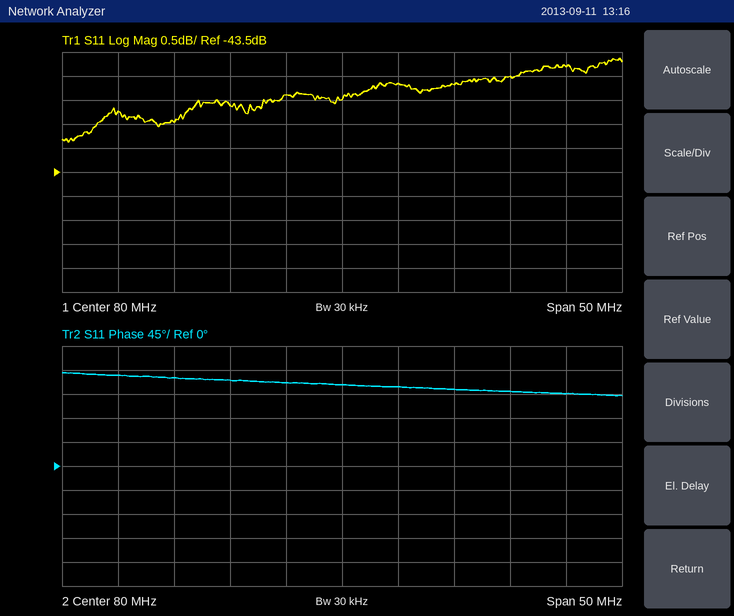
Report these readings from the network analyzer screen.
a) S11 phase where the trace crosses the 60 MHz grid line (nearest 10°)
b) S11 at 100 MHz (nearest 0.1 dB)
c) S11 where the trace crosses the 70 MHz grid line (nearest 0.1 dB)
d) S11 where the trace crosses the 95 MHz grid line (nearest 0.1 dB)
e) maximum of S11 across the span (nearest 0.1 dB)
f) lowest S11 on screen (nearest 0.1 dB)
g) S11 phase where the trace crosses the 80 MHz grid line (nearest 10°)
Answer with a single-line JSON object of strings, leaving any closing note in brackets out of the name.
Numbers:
{"S11 phase where the trace crosses the 60 MHz grid line": "170°", "S11 at 100 MHz": "-41.3 dB", "S11 where the trace crosses the 70 MHz grid line": "-42.1 dB", "S11 where the trace crosses the 95 MHz grid line": "-41.5 dB", "maximum of S11 across the span": "-41.1 dB", "lowest S11 on screen": "-42.9 dB", "S11 phase where the trace crosses the 80 MHz grid line": "150°"}
